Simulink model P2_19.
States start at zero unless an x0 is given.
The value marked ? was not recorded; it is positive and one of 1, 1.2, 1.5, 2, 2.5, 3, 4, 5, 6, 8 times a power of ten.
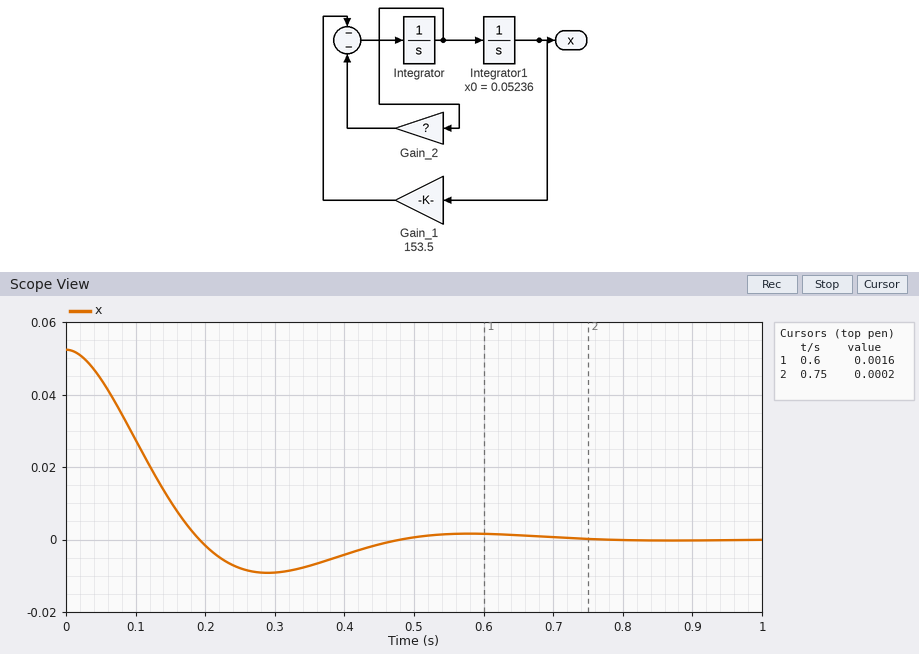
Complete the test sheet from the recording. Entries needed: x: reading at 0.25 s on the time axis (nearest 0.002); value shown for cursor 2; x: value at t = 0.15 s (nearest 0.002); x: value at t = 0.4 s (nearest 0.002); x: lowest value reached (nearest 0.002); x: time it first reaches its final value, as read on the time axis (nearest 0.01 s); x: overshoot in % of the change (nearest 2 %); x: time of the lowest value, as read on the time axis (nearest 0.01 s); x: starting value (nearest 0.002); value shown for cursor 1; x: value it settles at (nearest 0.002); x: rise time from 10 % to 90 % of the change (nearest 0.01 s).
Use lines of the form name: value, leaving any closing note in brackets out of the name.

x: reading at 0.25 s on the time axis: -0.008
value shown for cursor 2: 0.0002
x: value at t = 0.15 s: 0.010
x: value at t = 0.4 s: -0.004
x: lowest value reached: -0.010
x: time it first reaches its final value, as read on the time axis: 0.19 s
x: overshoot in % of the change: 18 %
x: time of the lowest value, as read on the time axis: 0.29 s
x: starting value: 0.052
value shown for cursor 1: 0.0016
x: value it settles at: 0.000
x: rise time from 10 % to 90 % of the change: 0.13 s
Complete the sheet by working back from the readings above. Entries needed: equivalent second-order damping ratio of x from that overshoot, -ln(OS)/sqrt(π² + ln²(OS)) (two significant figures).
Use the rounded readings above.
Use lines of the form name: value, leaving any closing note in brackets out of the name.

equivalent second-order damping ratio of x from that overshoot, -ln(OS)/sqrt(π² + ln²(OS)): 0.48
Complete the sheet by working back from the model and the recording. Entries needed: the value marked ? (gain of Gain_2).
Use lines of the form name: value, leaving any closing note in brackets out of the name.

the value marked ?: 12
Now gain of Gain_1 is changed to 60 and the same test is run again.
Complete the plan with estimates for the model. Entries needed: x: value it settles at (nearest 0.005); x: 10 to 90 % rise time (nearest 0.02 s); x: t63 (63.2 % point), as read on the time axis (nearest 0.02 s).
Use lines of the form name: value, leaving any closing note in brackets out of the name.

x: value it settles at: 0.000
x: 10 to 90 % rise time: 0.30 s
x: t63 (63.2 % point), as read on the time axis: 0.24 s
